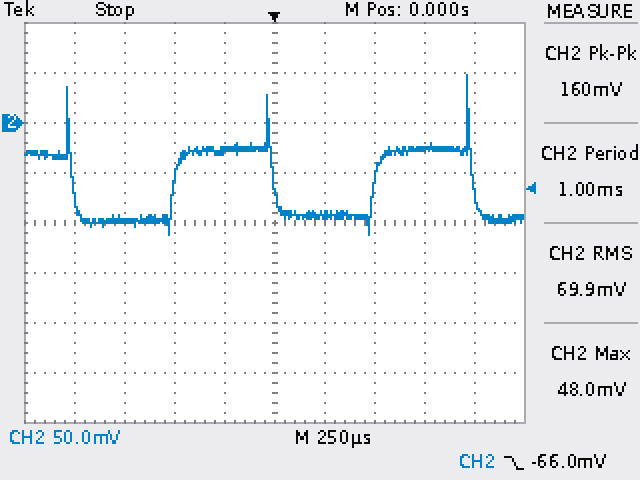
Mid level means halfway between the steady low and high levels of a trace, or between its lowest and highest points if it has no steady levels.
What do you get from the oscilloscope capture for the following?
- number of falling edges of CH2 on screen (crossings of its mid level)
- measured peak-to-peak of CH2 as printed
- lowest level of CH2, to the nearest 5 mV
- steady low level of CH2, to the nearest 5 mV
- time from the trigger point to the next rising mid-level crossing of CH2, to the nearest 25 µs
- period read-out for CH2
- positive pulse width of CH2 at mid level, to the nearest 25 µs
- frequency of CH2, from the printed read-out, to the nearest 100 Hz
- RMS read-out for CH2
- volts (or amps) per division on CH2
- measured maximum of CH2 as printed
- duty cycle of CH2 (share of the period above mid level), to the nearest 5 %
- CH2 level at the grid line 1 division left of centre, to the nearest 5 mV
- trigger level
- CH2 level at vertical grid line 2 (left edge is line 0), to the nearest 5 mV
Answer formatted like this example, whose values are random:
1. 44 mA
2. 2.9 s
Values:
1. 3
2. 160 mV
3. -110 mV
4. -95 mV
5. 500 µs
6. 1.00 ms
7. 500 µs
8. 1.0 kHz
9. 69.9 mV
10. 50 mV
11. 48.0 mV
12. 50 %
13. -30 mV
14. -66.0 mV
15. -100 mV
